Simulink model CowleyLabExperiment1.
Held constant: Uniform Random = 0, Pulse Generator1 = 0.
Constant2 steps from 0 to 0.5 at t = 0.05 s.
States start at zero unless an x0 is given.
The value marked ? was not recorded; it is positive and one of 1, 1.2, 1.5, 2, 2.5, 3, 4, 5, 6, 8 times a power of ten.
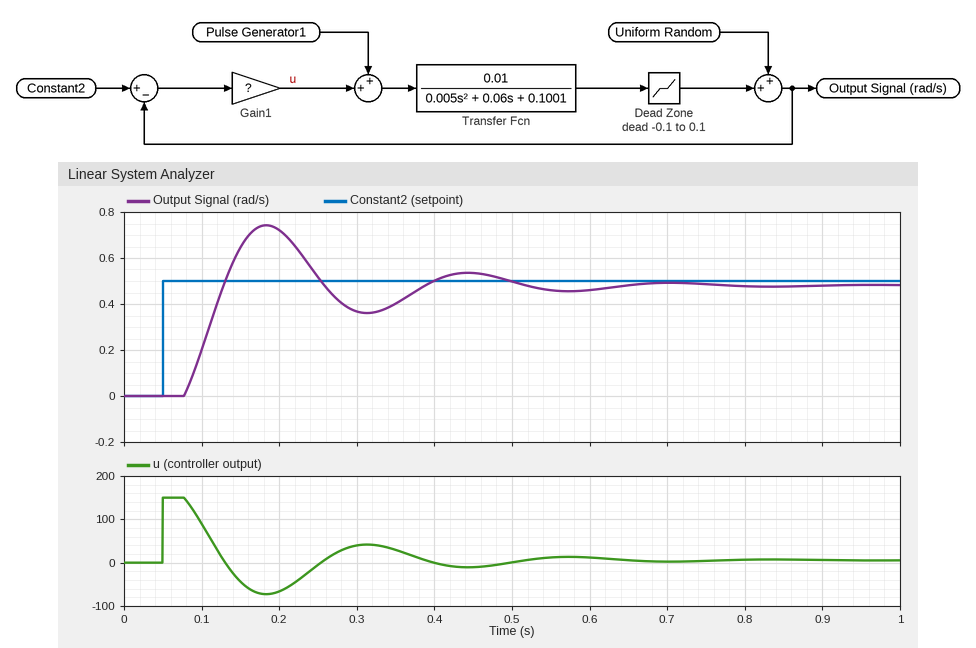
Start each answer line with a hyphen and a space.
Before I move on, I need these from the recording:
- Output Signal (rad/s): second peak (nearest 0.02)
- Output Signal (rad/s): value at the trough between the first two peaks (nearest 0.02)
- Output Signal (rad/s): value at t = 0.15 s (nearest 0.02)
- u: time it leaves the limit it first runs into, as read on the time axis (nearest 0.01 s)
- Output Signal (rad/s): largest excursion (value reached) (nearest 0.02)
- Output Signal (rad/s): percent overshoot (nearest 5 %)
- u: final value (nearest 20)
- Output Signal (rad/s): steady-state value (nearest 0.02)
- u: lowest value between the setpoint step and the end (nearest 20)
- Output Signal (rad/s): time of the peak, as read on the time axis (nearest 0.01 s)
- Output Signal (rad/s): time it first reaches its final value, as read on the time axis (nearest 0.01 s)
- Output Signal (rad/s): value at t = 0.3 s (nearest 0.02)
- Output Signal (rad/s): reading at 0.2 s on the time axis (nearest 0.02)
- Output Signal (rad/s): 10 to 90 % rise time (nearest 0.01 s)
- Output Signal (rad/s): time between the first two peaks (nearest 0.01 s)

- 0.54
- 0.36
- 0.64
- 0.08 s
- 0.74
- 55 %
- 0
- 0.48
- -80
- 0.18 s
- 0.13 s
- 0.36
- 0.72
- 0.04 s
- 0.26 s
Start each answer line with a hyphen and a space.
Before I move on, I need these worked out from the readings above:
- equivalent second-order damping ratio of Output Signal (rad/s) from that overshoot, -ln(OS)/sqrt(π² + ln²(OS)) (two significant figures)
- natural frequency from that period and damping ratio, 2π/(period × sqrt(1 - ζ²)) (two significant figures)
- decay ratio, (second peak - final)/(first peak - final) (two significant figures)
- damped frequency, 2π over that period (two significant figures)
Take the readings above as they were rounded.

- 0.19
- 25 rad/s
- 0.23
- 24 rad/s
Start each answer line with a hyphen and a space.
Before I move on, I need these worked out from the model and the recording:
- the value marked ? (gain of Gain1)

- 300
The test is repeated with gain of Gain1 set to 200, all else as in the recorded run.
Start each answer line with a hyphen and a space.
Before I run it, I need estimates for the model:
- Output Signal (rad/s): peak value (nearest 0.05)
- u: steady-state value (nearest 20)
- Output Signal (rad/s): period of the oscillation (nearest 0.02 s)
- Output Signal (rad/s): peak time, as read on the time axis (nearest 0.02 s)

- 0.70
- 0
- 0.32 s
- 0.22 s
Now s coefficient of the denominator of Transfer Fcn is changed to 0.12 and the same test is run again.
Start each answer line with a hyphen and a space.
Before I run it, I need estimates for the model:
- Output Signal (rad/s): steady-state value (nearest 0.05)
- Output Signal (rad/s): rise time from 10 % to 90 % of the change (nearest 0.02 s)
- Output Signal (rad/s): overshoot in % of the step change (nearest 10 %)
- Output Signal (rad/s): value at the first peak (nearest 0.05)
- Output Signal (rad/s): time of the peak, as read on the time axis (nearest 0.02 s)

- 0.50
- 0.06 s
- 20 %
- 0.60
- 0.20 s
